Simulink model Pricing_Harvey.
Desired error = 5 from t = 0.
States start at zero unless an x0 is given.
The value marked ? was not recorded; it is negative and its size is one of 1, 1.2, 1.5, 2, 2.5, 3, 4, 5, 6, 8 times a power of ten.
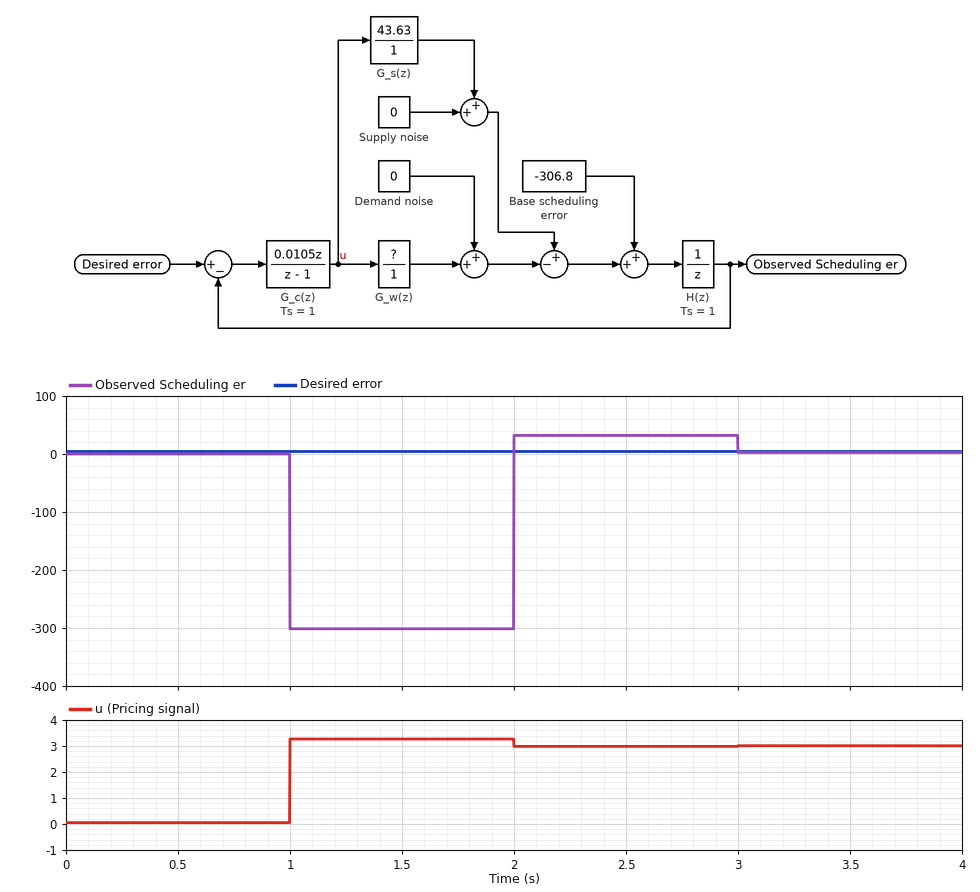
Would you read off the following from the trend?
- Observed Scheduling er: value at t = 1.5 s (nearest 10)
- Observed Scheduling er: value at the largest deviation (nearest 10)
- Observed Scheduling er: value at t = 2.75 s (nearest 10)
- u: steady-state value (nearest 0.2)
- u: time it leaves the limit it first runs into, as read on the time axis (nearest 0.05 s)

-300
-300
30
3.0
1.00 s
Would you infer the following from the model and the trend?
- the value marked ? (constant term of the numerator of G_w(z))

-60
